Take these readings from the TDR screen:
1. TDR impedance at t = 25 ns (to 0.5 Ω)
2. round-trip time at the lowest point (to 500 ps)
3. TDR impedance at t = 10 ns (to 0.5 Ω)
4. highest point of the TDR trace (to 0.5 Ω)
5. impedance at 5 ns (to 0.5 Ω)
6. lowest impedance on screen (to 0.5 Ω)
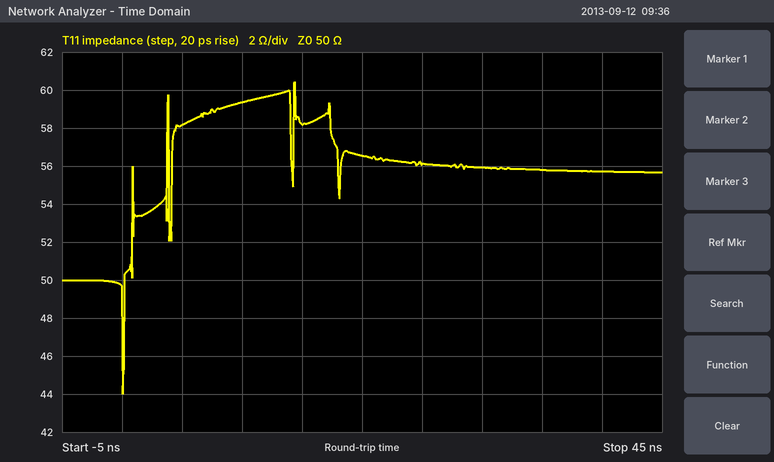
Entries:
56.0 Ω
0.0 ns
59.5 Ω
60.5 Ω
58.0 Ω
44.0 Ω
